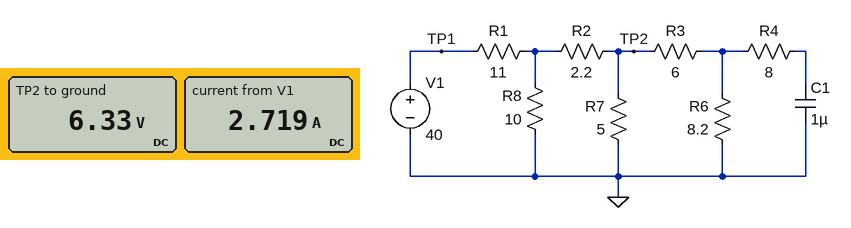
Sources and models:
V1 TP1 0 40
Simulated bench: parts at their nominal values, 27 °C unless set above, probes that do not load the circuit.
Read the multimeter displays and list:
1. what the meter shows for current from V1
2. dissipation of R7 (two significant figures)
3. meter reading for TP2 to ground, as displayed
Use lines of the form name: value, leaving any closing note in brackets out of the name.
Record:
what the meter shows for current from V1: 2.719 A
dissipation of R7: 8.0 W
meter reading for TP2 to ground, as displayed: 6.33 V
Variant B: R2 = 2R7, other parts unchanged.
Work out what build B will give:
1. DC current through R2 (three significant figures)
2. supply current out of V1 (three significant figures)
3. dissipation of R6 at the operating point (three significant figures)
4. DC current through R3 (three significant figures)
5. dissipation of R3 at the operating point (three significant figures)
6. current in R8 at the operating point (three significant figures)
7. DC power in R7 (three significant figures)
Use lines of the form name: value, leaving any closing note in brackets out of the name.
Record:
DC current through R2: 1.64 A
supply current out of V1: 2.68 A
dissipation of R6 at the operating point: 1.49 W
DC current through R3: 426 mA
dissipation of R3 at the operating point: 1.09 W
current in R8 at the operating point: 1.05 A
DC power in R7: 7.33 W
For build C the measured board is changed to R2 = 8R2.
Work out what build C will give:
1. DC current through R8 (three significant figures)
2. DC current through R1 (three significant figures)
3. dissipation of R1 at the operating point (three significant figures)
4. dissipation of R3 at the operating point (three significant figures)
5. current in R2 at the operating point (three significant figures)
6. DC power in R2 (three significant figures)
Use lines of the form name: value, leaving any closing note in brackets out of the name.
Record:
DC current through R8: 1.32 A
DC current through R1: 2.43 A
dissipation of R1 at the operating point: 65.2 W
dissipation of R3 at the operating point: 503 mW
current in R2 at the operating point: 1.11 A
DC power in R2: 10.1 W
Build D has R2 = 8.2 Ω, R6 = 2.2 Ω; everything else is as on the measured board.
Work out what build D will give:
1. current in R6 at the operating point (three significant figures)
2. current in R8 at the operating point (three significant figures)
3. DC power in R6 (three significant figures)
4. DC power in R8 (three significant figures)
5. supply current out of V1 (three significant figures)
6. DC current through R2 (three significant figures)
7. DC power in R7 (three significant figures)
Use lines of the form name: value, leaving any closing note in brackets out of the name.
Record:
current in R6 at the operating point: 436 mA
current in R8 at the operating point: 1.30 A
DC power in R6: 418 mW
DC power in R8: 16.9 W
supply current out of V1: 2.45 A
DC current through R2: 1.15 A
DC power in R7: 2.56 W
